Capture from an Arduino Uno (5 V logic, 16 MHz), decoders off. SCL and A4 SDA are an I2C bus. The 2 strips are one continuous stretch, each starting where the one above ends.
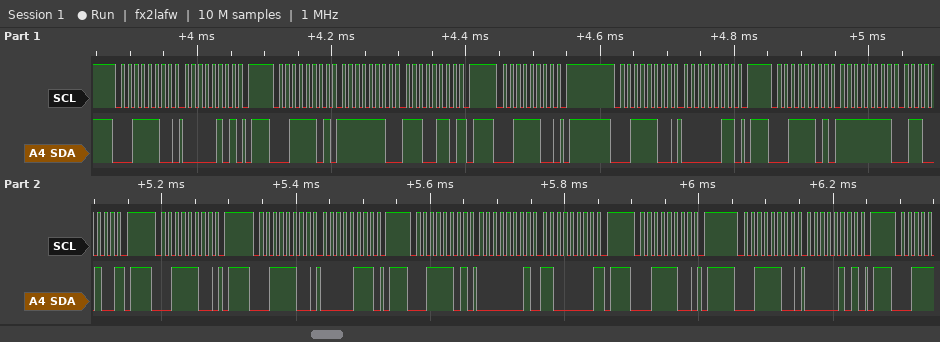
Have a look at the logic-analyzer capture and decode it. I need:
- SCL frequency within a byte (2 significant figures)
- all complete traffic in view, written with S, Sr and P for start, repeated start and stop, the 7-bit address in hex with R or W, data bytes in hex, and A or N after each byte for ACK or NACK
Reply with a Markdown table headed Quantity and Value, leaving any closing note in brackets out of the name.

| Quantity | Value |
|---|---|
| SCL frequency within a byte | 100 kHz |
| all complete traffic in view, written with S, Sr and P for start, repeated start and stop, the 7-bit address in hex with R or W, data bytes in hex, and A or N after each byte for ACK or NACK | S 1EW A 05 A P S 1ER A FE A E6 N P S 1EW A P S 1EW A 03 A P S 1ER A FF A 64 N P S 1EW A P S 1EW A 07 A P S 1ER A 01 A C0 N P S 1EW A P S 1EW A 05 A P |
